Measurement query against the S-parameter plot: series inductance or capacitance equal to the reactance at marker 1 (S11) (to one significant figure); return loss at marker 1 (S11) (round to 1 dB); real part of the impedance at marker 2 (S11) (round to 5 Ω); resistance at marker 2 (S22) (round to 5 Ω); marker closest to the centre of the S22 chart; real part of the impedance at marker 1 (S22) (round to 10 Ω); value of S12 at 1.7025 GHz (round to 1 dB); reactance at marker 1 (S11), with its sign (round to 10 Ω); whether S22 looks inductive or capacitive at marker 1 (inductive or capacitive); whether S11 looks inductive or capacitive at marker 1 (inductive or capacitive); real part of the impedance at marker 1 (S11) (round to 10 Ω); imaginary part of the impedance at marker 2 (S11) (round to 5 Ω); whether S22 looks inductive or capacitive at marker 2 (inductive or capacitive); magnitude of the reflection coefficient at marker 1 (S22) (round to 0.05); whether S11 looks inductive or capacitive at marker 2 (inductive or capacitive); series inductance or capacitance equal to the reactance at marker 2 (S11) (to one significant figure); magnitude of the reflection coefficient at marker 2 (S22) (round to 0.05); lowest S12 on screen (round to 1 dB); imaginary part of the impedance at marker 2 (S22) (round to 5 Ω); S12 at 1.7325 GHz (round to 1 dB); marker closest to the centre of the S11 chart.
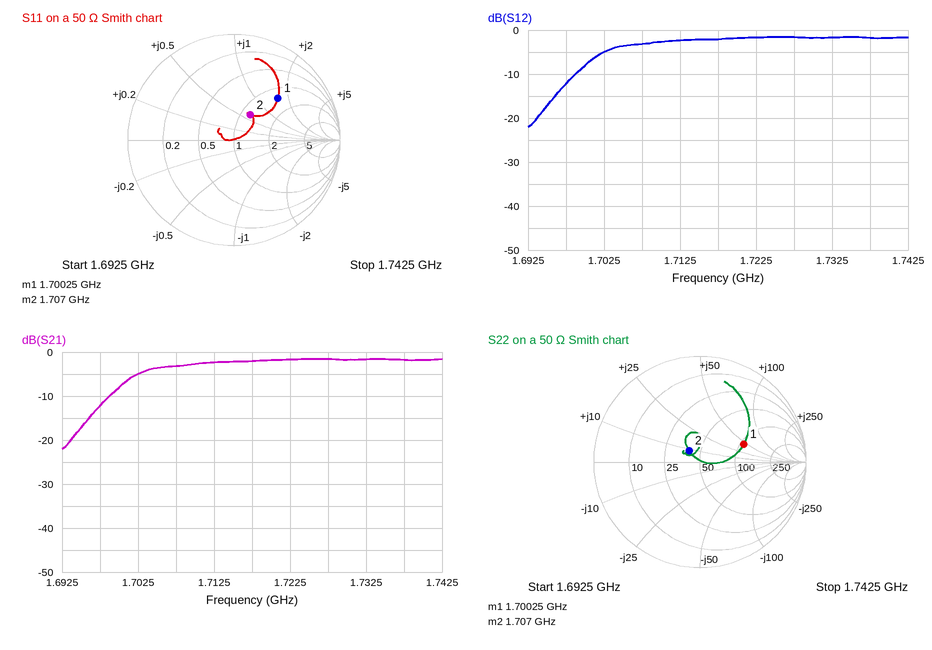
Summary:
7 nH
5 dB
60 Ω
40 Ω
marker 2
110 Ω
-5 dB
+80 Ω
inductive
inductive
70 Ω
+30 Ω
inductive
0.45
inductive
3 nH
0.15
-22 dB
+10 Ω
-2 dB
marker 2
